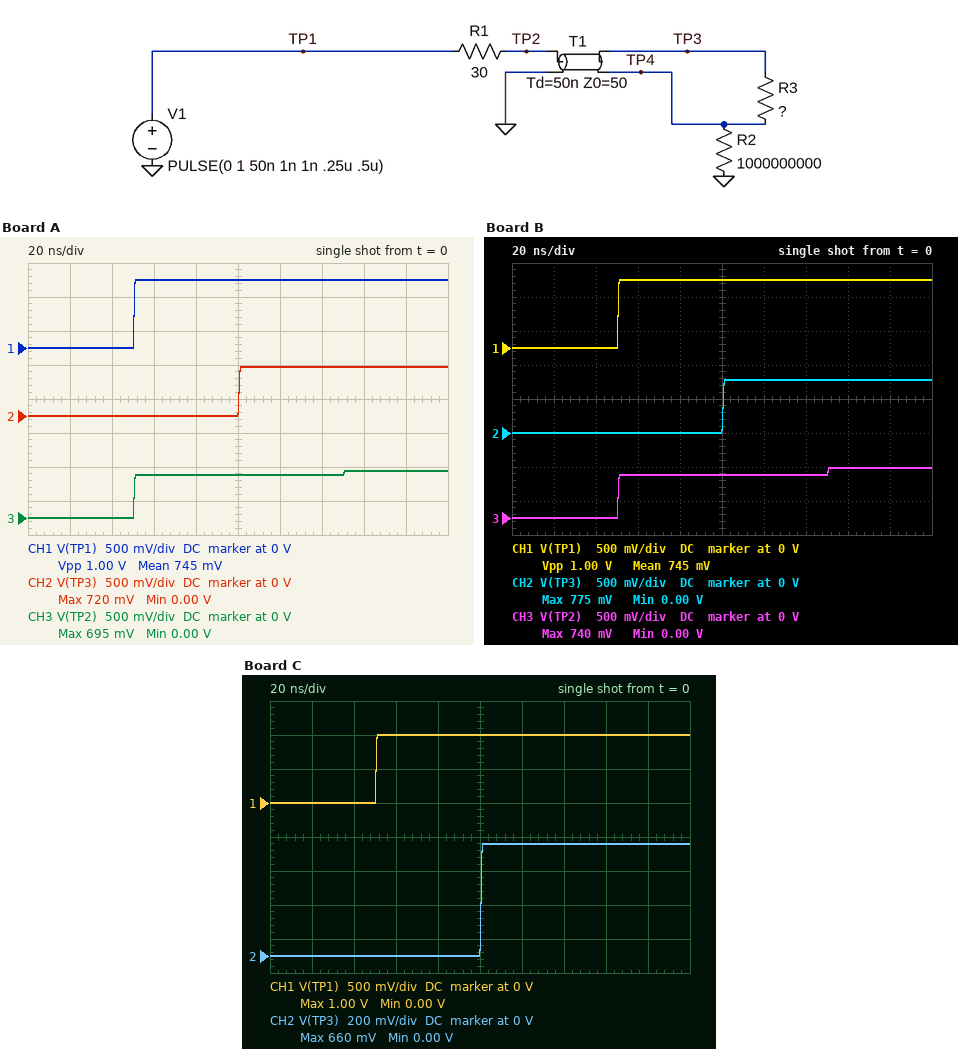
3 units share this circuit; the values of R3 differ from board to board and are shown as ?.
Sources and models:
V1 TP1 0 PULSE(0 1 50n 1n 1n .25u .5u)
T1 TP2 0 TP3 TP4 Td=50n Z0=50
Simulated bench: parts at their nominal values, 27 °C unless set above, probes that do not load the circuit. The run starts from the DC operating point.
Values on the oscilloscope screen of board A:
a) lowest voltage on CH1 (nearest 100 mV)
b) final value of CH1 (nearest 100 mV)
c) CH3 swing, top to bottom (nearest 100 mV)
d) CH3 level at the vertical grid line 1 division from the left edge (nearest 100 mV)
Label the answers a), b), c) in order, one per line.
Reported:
a) 0 V
b) 1.0 V
c) 700 mV
d) 0 V
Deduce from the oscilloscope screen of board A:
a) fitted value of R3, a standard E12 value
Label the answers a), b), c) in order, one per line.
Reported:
a) 68 Ω
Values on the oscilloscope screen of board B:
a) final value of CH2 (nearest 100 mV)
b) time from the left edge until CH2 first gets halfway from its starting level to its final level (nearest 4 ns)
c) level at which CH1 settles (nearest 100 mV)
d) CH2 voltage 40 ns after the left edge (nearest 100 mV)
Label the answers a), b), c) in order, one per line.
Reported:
a) 800 mV
b) 100 ns
c) 1.0 V
d) 0 V
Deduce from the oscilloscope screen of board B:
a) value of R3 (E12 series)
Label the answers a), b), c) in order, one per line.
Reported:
a) 82 Ω
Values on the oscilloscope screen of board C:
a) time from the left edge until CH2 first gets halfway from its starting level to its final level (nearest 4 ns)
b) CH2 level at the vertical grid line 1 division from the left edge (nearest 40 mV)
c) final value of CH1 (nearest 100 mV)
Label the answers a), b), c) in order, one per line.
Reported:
a) 100 ns
b) 0 V
c) 1.0 V
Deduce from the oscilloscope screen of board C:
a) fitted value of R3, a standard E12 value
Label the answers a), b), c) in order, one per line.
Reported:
a) 56 Ω
